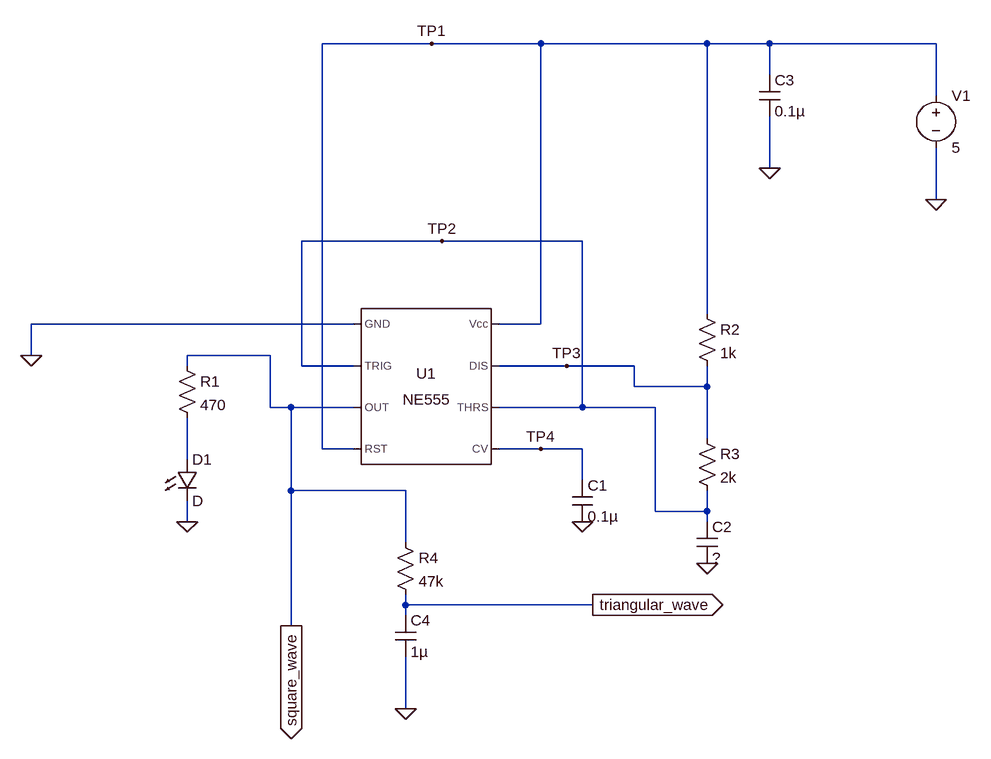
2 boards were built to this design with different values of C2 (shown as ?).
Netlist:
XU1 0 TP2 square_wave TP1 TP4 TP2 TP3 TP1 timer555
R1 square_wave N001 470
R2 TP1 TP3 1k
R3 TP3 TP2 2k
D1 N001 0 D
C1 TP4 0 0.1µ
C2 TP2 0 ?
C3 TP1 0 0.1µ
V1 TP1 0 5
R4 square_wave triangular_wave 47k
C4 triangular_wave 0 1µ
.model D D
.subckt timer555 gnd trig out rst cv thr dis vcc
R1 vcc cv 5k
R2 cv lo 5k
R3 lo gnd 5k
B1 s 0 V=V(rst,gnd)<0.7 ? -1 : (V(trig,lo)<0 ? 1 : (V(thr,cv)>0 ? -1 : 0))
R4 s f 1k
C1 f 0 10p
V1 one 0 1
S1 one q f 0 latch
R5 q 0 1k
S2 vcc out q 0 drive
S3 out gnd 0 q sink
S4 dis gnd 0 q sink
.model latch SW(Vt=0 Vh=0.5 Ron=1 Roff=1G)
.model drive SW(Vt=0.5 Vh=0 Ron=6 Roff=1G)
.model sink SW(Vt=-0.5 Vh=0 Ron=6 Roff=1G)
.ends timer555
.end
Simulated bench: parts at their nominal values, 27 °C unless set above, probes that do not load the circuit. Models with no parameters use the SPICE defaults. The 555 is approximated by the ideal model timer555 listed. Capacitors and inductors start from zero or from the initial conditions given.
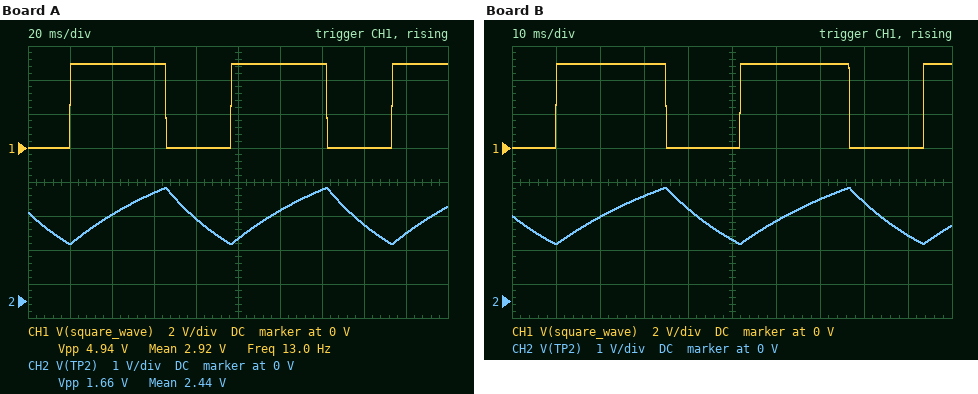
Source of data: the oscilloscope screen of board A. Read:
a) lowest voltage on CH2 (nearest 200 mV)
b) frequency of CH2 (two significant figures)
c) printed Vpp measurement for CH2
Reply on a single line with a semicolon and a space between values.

1.6 V; 13 Hz; 1.66 V
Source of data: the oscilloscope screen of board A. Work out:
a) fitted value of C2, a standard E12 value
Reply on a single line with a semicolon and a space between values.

22 µF
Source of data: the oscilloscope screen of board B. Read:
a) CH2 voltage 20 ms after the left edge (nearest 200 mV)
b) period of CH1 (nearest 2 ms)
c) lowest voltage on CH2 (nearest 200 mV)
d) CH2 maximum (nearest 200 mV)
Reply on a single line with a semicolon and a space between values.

2.4 V; 42 ms; 1.6 V; 3.4 V
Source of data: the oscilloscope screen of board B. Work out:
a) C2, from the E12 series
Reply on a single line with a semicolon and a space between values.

12 µF
